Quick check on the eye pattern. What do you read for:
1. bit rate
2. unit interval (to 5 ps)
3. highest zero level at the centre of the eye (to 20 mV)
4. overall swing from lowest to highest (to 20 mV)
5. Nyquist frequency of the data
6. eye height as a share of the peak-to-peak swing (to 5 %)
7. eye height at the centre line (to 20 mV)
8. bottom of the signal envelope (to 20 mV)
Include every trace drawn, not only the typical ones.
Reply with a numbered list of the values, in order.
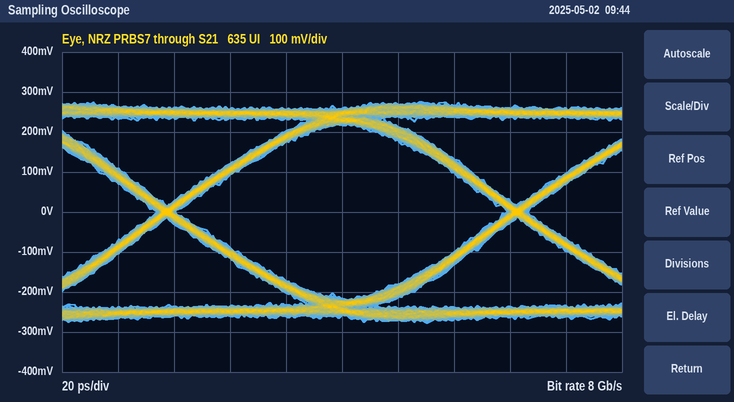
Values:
1. 8 Gb/s
2. 125 ps
3. -220 mV
4. 560 mV
5. 4 GHz
6. 80 %
7. 440 mV
8. -280 mV
